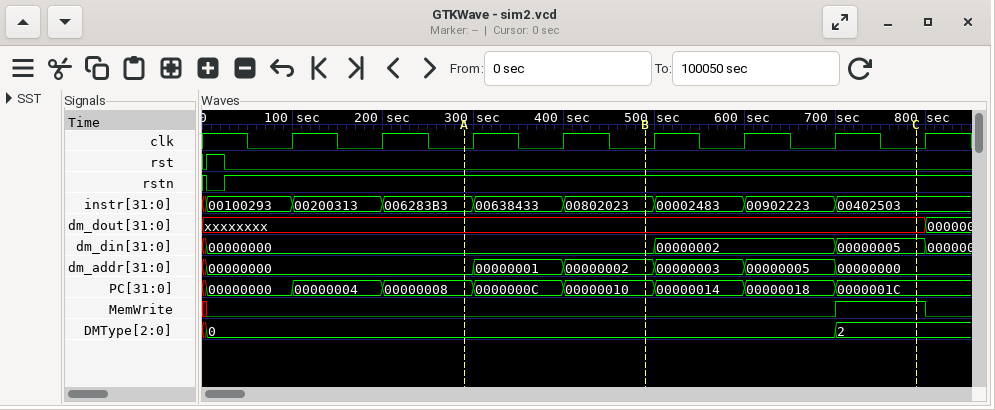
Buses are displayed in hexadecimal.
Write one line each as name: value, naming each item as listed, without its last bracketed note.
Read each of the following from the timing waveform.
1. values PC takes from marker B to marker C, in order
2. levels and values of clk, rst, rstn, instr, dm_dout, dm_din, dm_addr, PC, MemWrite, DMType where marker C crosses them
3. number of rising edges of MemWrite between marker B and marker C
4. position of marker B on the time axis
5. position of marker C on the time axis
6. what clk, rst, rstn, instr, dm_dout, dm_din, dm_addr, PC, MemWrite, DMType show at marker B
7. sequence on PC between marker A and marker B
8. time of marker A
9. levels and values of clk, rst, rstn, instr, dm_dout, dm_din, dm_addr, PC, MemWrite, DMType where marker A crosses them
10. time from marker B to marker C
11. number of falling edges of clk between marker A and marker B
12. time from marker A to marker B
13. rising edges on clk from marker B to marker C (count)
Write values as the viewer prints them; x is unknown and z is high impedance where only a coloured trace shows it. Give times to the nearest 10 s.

values PC takes from marker B to marker C, in order: 00000010, 00000014, 00000018, 0000001C
levels and values of clk, rst, rstn, instr, dm_dout, dm_din, dm_addr, PC, MemWrite, DMType where marker C crosses them: clk=0, rst=0, rstn=1, instr=00402503, dm_dout=xxxxxxxx, dm_din=00000005, dm_addr=00000000, PC=0000001C, MemWrite=1, DMType=2
number of rising edges of MemWrite between marker B and marker C: 1
position of marker B on the time axis: 490 s
position of marker C on the time axis: 790 s
what clk, rst, rstn, instr, dm_dout, dm_din, dm_addr, PC, MemWrite, DMType show at marker B: clk=0, rst=0, rstn=1, instr=00802023, dm_dout=xxxxxxxx, dm_din=00000000, dm_addr=00000002, PC=00000010, MemWrite=0, DMType=0
sequence on PC between marker A and marker B: 00000008, 0000000C, 00000010
time of marker A: 290 s
levels and values of clk, rst, rstn, instr, dm_dout, dm_din, dm_addr, PC, MemWrite, DMType where marker A crosses them: clk=0, rst=0, rstn=1, instr=006283B3, dm_dout=xxxxxxxx, dm_din=00000000, dm_addr=00000000, PC=00000008, MemWrite=0, DMType=0
time from marker B to marker C: 300 s
number of falling edges of clk between marker A and marker B: 2
time from marker A to marker B: 200 s
rising edges on clk from marker B to marker C: 3
